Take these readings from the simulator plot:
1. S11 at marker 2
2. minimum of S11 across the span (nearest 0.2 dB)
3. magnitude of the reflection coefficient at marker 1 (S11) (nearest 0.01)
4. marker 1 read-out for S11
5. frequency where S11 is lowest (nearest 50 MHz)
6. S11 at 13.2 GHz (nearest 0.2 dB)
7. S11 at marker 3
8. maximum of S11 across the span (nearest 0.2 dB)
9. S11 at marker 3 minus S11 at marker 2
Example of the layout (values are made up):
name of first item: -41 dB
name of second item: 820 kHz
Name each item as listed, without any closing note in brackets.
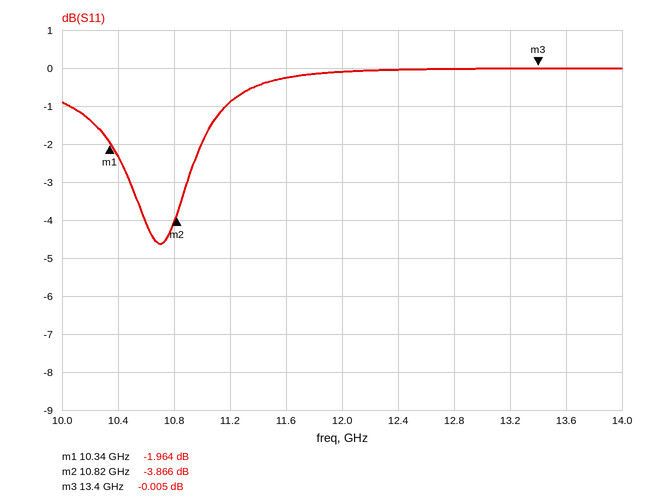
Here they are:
S11 at marker 2: -3.866 dB
minimum of S11 across the span: -4.6 dB
magnitude of the reflection coefficient at marker 1 (S11): 0.80
marker 1 read-out for S11: -1.964 dB
frequency where S11 is lowest: 10.70 GHz
S11 at 13.2 GHz: 0.0 dB
S11 at marker 3: -0.005 dB
maximum of S11 across the span: 0.0 dB
S11 at marker 3 minus S11 at marker 2: 3.861 dB
